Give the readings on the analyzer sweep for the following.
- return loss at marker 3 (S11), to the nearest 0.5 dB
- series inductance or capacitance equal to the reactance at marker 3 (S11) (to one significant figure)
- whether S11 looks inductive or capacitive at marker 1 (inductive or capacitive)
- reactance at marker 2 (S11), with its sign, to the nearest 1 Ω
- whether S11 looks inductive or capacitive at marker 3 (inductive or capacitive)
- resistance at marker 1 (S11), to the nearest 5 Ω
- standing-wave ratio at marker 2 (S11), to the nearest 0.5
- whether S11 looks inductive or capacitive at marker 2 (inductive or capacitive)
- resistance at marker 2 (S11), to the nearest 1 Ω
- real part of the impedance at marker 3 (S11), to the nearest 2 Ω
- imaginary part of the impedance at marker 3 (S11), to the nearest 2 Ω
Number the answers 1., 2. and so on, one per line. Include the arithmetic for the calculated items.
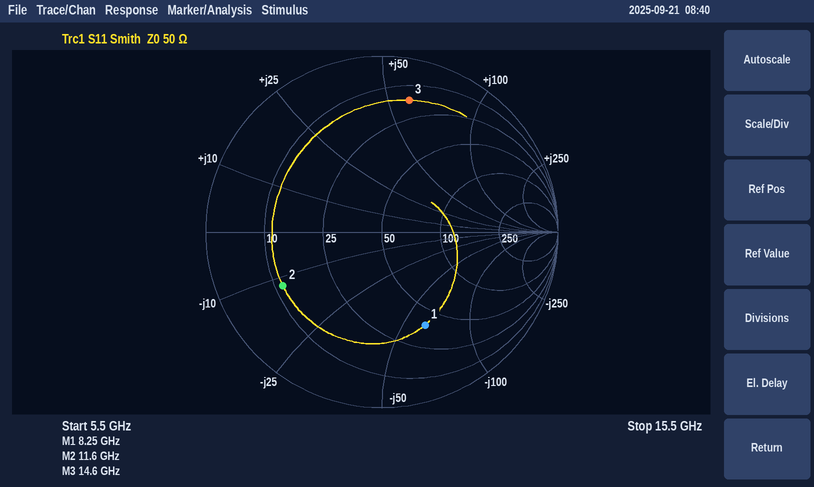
1. 2.5 dB
2. L = 58 Ω/(2π × 14.6 GHz) ≈ 632 pH, so 600 pH to one significant figure
3. capacitive
4. -12 Ω
5. inductive
6. 40 Ω
7. 4.5
8. capacitive
9. 12 Ω
10. 16 Ω
11. +58 Ω
